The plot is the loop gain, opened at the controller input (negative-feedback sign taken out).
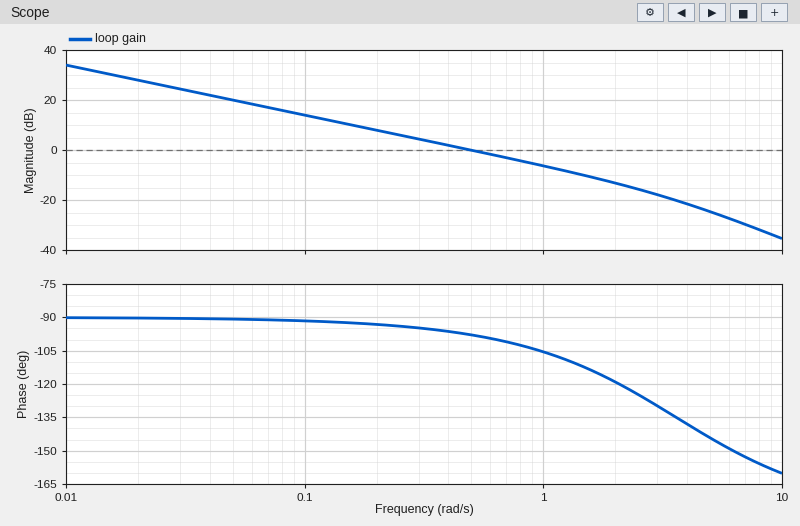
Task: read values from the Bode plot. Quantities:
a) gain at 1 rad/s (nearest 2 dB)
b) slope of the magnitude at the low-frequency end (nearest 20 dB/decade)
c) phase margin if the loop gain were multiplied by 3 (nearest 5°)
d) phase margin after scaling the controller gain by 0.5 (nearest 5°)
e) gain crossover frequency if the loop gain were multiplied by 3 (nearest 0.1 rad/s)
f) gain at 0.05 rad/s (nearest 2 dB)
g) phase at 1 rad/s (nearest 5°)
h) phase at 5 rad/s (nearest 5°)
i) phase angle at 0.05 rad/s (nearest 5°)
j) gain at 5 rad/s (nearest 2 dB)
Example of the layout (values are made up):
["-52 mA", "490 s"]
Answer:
["-6 dB", "-20 dB/decade", "70°", "85°", "1.4 rad/s", "20 dB", "-105°", "-145°", "-90°", "-24 dB"]
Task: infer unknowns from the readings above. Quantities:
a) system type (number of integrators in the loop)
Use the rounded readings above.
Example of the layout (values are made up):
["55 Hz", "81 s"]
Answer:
["1"]
